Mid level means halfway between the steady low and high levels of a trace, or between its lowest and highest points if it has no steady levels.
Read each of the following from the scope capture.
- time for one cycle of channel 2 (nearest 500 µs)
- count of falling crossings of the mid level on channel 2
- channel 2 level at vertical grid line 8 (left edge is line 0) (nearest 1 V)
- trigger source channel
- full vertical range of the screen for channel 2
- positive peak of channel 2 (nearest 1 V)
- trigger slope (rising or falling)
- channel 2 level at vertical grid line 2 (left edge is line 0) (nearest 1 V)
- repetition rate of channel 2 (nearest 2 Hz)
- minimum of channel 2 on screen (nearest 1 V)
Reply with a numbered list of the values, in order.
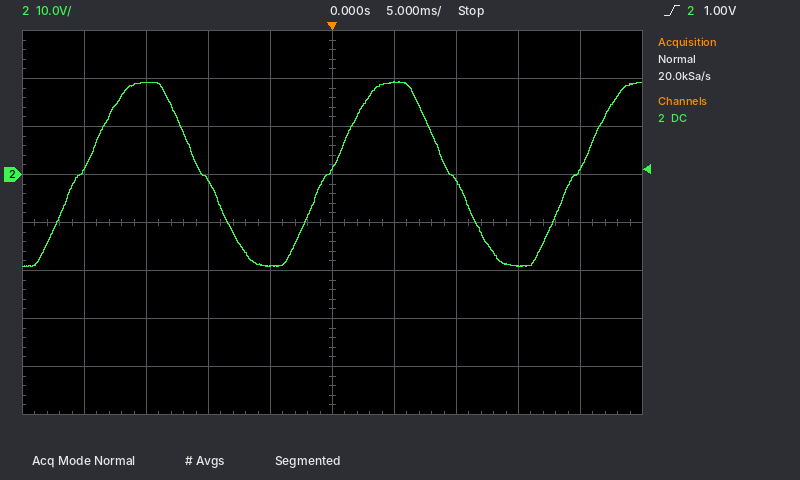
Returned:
1. 20.0 ms
2. 2
3. -19 V
4. channel 2
5. 80 V
6. 19 V
7. rising
8. 19 V
9. 50 Hz
10. -19 V
